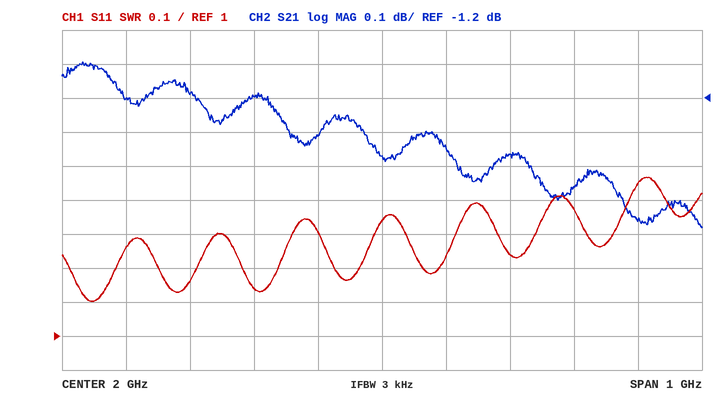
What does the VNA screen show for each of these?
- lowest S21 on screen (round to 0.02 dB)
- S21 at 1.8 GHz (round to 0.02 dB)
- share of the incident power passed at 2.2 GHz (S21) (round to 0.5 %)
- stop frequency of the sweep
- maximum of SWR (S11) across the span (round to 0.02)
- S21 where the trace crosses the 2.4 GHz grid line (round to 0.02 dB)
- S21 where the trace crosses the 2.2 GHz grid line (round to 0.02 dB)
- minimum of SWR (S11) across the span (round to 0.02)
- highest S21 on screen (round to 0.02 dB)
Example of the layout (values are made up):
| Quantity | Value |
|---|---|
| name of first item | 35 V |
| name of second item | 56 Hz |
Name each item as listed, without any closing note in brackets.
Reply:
| Quantity | Value |
|---|---|
| lowest S21 on screen | -1.58 dB |
| S21 at 1.8 GHz | -1.20 dB |
| share of the incident power passed at 2.2 GHz (S21) | 73.0 % |
| stop frequency of the sweep | 2.5 GHz |
| maximum of SWR (S11) across the span | 1.46 |
| S21 where the trace crosses the 2.4 GHz grid line | -1.56 dB |
| S21 where the trace crosses the 2.2 GHz grid line | -1.36 dB |
| minimum of SWR (S11) across the span | 1.10 |
| highest S21 on screen | -1.10 dB |
